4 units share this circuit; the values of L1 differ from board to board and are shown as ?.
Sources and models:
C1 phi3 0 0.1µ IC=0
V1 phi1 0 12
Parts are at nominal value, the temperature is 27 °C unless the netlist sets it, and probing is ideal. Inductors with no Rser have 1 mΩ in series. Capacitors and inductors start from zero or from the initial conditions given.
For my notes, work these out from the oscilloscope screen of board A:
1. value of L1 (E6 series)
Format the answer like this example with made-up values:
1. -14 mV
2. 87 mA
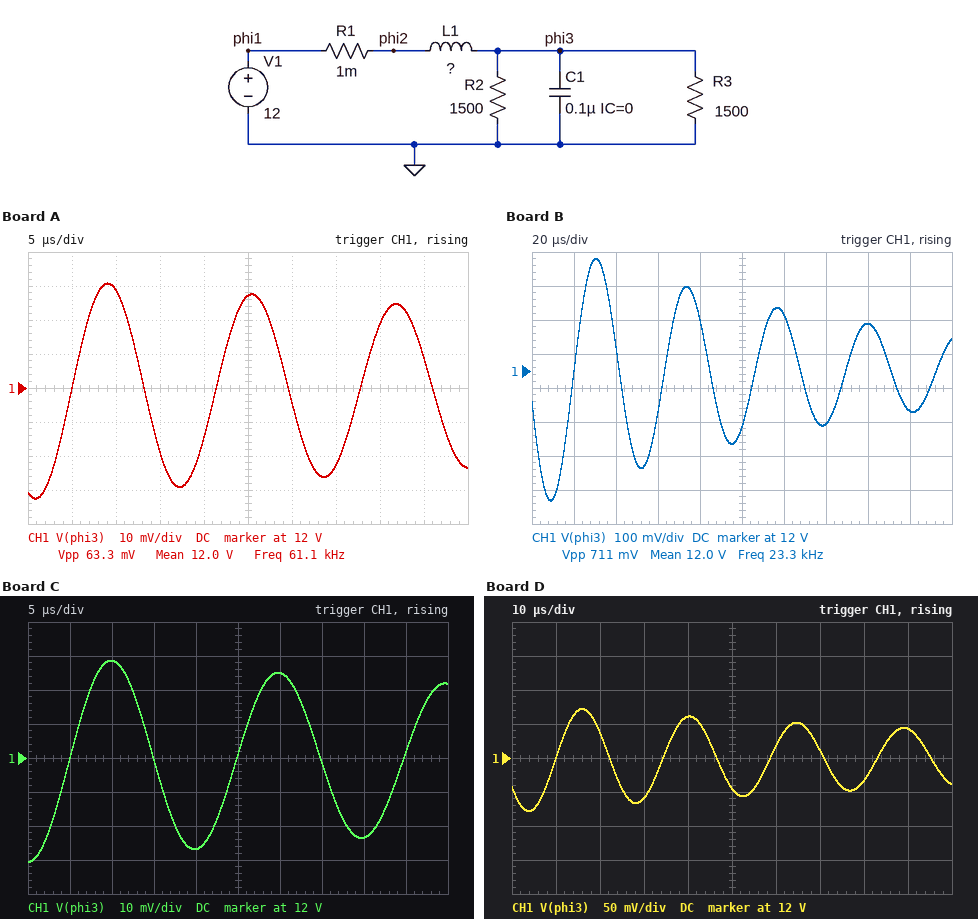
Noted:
1. 68 µH
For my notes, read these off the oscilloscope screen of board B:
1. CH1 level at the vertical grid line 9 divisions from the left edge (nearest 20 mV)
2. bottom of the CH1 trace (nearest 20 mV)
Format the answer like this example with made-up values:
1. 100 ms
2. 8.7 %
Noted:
1. 11.88 V
2. 11.62 V
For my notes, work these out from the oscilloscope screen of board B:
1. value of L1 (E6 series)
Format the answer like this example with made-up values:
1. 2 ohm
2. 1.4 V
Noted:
1. 470 µH
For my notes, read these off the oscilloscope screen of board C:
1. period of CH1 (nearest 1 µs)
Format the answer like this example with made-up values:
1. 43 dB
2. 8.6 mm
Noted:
1. 20 µs
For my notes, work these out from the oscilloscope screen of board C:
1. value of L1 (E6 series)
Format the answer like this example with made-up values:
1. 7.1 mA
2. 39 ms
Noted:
1. 100 µH
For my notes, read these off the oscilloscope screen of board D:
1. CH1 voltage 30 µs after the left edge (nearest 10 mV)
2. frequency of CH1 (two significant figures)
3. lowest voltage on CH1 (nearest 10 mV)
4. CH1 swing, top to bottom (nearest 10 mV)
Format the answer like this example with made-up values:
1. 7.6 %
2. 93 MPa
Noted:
1. 11.94 V
2. 41 kHz
3. 11.92 V
4. 150 mV
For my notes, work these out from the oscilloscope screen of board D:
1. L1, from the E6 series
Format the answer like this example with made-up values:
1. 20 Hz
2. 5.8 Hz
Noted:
1. 150 µH
